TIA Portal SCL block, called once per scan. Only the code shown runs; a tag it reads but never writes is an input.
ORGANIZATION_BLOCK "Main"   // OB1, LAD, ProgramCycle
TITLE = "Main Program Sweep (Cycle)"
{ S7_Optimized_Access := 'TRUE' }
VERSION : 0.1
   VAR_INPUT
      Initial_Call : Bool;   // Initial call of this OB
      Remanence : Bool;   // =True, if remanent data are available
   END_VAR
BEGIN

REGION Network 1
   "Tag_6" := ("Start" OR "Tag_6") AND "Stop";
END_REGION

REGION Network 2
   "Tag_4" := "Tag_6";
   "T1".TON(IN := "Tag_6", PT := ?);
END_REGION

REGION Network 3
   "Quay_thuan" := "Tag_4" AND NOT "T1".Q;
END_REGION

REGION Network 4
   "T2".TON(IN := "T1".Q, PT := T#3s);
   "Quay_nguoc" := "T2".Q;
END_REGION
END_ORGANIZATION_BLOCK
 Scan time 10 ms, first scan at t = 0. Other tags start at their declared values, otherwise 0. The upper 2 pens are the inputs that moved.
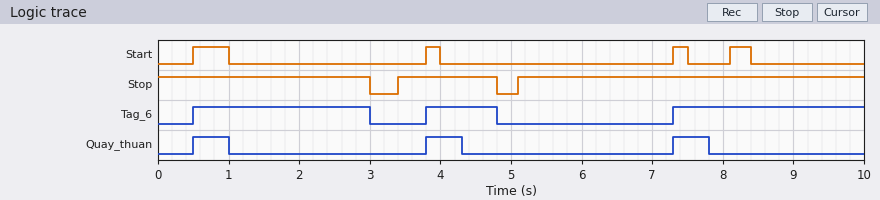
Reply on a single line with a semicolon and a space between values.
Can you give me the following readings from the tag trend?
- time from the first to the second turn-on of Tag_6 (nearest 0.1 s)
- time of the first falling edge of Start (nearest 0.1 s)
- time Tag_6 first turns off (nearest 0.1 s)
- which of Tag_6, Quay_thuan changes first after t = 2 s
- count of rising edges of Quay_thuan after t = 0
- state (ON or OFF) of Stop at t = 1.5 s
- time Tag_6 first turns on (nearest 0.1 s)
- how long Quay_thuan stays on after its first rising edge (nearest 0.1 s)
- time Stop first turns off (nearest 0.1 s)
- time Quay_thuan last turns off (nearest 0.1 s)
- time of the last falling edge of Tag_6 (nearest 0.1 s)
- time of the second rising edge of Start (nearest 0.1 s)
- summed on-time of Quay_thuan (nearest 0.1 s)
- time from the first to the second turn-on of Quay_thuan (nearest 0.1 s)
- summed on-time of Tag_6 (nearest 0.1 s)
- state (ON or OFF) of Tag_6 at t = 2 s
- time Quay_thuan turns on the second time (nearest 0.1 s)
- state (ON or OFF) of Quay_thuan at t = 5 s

3.3 s; 1.0 s; 3.0 s; Tag_6; 3; ON; 0.5 s; 0.5 s; 3.0 s; 7.8 s; 4.8 s; 3.8 s; 1.5 s; 3.3 s; 6.2 s; ON; 3.8 s; OFF
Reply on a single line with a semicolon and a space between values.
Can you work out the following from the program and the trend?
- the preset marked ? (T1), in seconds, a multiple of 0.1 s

0.5 s
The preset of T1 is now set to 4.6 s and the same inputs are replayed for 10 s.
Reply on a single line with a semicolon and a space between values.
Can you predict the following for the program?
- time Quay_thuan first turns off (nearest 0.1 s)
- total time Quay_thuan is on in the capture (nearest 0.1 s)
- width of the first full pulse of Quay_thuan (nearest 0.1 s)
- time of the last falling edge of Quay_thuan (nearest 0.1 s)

3.0 s; 6.2 s; 2.5 s; 4.8 s
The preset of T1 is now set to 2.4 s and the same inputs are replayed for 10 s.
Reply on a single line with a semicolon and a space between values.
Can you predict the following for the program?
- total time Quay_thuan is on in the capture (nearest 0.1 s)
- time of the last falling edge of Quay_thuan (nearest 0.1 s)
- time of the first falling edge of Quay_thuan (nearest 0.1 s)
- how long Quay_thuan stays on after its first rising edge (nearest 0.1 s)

5.8 s; 9.7 s; 2.9 s; 2.4 s
